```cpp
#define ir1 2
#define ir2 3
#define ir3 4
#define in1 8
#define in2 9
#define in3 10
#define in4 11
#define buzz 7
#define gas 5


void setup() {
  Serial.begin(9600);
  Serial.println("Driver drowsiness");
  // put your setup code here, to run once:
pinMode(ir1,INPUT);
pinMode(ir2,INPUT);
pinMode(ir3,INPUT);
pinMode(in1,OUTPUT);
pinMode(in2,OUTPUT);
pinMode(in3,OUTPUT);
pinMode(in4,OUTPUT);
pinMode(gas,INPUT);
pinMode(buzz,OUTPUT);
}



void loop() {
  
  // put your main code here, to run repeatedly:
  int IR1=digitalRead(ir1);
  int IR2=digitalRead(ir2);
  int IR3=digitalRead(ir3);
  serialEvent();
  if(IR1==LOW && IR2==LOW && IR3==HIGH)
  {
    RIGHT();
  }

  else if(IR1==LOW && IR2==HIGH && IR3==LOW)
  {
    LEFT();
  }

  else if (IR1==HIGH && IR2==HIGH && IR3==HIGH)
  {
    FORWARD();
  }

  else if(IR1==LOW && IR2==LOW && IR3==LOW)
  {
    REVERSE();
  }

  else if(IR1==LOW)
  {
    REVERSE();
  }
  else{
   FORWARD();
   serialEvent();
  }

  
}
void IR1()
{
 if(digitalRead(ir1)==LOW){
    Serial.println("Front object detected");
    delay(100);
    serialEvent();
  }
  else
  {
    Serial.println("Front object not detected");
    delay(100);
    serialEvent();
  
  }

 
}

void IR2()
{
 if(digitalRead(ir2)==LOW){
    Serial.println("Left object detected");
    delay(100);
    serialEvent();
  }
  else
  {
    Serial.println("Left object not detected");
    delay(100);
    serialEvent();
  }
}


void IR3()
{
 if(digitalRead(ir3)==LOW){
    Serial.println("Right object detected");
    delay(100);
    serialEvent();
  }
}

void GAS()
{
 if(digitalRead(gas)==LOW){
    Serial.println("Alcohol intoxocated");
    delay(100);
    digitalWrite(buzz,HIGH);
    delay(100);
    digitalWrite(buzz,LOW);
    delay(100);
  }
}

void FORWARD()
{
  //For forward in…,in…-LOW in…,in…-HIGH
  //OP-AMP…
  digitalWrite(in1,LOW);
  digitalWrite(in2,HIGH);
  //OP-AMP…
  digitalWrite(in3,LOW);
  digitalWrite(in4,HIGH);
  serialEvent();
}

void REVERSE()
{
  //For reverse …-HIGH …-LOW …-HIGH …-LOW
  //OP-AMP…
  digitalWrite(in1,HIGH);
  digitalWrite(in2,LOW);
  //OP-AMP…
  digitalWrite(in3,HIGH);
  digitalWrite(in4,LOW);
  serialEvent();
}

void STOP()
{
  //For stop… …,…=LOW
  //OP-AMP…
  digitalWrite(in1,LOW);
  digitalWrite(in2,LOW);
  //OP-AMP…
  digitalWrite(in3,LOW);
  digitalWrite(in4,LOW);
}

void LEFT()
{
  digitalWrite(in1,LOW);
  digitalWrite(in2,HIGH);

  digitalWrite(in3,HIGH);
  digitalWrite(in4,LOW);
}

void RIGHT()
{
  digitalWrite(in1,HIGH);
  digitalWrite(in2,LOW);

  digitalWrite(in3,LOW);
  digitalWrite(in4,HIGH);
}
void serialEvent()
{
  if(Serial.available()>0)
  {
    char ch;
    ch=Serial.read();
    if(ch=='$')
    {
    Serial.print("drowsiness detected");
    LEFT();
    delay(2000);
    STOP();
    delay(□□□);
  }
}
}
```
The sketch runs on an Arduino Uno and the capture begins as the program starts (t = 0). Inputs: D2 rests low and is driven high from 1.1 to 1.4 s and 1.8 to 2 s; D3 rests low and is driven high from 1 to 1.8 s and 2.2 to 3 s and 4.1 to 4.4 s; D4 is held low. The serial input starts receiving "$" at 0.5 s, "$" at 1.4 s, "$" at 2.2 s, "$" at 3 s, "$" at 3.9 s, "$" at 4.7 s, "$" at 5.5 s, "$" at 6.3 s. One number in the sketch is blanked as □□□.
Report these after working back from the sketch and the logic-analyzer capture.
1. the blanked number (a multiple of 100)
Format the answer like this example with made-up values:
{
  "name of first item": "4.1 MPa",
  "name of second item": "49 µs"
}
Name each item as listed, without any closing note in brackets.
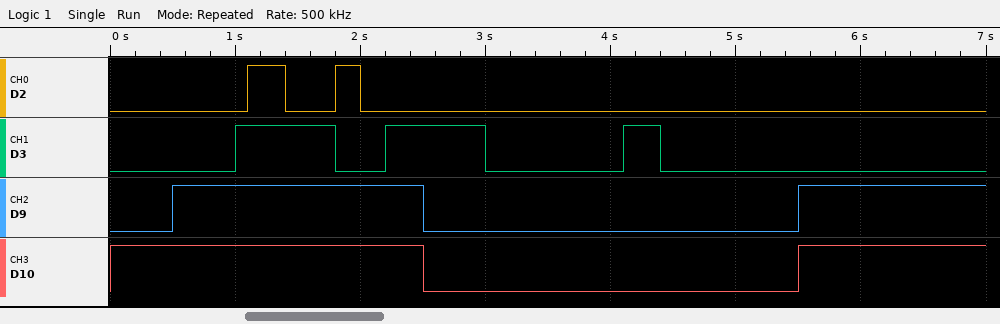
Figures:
{
  "the blanked number": "3000"
}
